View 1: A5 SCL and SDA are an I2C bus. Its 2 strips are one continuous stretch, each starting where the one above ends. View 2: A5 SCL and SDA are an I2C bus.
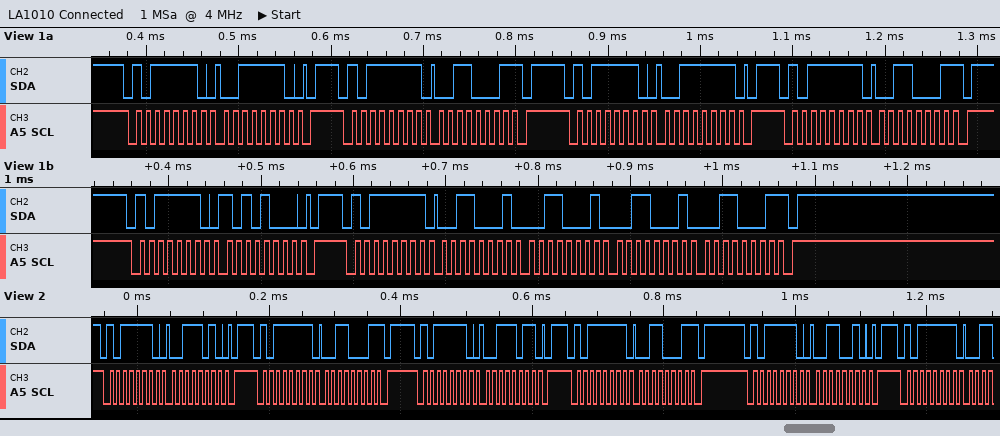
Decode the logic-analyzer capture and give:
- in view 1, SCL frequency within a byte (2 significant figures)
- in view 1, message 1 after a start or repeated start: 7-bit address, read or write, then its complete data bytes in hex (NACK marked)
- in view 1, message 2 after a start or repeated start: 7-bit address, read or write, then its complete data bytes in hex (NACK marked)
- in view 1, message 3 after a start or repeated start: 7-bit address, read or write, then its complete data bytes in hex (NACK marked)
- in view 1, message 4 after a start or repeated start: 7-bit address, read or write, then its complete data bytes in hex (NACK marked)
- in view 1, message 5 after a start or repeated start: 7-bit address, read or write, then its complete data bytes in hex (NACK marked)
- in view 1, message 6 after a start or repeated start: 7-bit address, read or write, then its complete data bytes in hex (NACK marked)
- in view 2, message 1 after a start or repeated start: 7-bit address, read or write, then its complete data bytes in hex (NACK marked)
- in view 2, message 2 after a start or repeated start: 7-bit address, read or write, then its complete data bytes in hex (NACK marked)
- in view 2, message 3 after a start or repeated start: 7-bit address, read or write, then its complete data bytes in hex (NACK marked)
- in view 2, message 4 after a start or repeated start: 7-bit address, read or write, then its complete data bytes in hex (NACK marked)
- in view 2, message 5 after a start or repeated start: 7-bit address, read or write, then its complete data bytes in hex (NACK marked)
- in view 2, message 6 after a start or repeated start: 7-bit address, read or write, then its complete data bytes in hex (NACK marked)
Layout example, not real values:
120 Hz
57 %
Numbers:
100 kHz
0x5F write: 3E
0x5F read: 31 NACK
0x5F write: 3F
0x5F read: 31 NACK
0x5F write: A8
0x5F read: 31 31 31 31 NACK
0x5F write: 3A
0x5F read: 31 NACK
0x5F write: 3B
0x5F read: 31 NACK
0x5F write: 32
0x5F read
